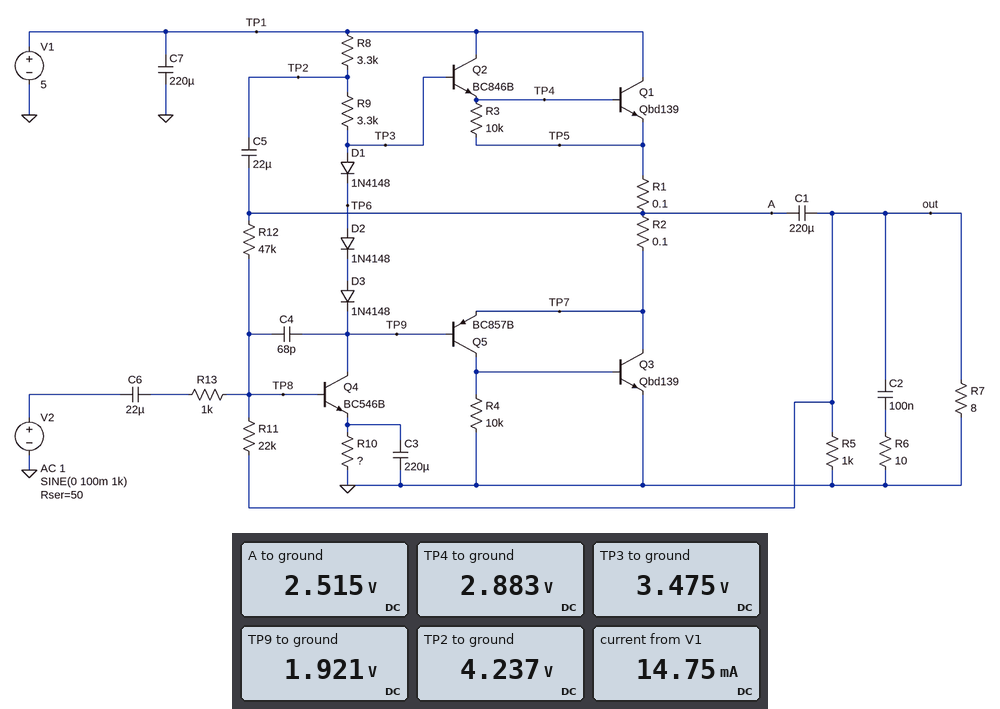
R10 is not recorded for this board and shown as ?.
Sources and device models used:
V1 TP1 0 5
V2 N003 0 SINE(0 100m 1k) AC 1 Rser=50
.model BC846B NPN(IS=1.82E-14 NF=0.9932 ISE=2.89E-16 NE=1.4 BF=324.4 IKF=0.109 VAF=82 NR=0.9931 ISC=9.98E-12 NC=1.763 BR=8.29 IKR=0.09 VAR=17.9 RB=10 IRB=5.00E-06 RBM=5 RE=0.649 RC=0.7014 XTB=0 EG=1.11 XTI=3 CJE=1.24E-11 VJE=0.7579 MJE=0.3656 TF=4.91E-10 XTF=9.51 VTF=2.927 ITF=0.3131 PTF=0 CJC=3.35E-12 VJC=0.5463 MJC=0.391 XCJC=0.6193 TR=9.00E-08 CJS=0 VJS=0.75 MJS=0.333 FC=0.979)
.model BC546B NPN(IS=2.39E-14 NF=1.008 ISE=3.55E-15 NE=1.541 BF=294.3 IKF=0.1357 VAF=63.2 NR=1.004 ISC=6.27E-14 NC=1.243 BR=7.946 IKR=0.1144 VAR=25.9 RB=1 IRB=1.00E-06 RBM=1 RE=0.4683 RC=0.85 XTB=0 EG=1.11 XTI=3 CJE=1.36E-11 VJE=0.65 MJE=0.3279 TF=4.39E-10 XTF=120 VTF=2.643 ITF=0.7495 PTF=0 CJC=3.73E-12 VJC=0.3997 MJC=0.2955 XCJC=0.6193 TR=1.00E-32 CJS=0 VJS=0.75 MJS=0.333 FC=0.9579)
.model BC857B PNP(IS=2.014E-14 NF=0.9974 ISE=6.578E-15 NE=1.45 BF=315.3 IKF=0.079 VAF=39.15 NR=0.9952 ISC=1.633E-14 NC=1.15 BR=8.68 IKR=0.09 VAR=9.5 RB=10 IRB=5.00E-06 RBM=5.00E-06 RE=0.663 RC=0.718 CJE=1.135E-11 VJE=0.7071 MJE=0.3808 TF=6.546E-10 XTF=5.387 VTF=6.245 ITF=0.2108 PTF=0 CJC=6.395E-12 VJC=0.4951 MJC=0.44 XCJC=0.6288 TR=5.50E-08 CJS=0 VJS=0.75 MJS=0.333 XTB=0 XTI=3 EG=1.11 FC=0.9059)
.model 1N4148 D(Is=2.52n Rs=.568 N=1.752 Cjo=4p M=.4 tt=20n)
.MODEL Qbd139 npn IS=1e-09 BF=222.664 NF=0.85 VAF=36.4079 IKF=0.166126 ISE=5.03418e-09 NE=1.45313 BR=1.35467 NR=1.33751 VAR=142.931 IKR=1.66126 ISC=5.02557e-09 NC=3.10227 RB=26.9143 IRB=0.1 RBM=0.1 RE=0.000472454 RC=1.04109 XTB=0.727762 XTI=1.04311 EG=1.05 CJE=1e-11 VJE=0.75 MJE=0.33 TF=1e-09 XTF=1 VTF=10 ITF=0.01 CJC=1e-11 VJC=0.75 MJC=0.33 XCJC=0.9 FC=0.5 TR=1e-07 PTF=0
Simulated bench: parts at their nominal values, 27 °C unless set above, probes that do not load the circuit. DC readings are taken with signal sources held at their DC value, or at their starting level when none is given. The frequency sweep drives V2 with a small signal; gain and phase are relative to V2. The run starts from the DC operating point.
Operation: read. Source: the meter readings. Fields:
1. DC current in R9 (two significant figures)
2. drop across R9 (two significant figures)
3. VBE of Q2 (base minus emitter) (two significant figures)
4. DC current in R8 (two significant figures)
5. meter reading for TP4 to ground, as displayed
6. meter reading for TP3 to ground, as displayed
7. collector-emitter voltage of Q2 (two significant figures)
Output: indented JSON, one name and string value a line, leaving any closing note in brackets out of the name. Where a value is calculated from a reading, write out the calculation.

{
  "DC current in R9": "(4.237 V - 3.475 V) / 3.3 kΩ = 230 µA",
  "drop across R9": "4.237 V - 3.475 V = 760 mV",
  "VBE of Q2 (base minus emitter)": "3.475 V - 2.883 V = 590 mV",
  "DC current in R8": "(5 V - 4.237 V) / 3.3 kΩ = 230 µA",
  "meter reading for TP4 to ground, as displayed": "2.883 V",
  "meter reading for TP3 to ground, as displayed": "3.475 V",
  "collector-emitter voltage of Q2": "5 V - 2.883 V = 2.1 V"
}
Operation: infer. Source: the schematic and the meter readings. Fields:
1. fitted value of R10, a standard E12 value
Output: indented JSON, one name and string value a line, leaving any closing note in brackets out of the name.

{
  "fitted value of R10, a standard E12 value": "820 Ω"
}
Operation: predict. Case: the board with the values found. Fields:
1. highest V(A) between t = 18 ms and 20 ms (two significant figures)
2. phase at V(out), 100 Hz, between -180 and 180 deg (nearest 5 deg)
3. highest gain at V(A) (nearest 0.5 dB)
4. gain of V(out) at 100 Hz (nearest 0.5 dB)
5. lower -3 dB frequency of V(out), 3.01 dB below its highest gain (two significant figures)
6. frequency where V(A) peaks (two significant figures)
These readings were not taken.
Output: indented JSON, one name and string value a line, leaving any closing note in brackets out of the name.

{
  "highest V(A) between t = 18 ms and 20 ms": "3.8 V",
  "phase at V(out), 100 Hz, between -180 and 180 deg": "-160 deg",
  "highest gain at V(A)": "31.0 dB",
  "gain of V(out) at 100 Hz": "22.0 dB",
  "lower -3 dB frequency of V(out), 3.01 dB below its highest gain": "28 Hz",
  "frequency where V(A) peaks": "17 Hz"
}
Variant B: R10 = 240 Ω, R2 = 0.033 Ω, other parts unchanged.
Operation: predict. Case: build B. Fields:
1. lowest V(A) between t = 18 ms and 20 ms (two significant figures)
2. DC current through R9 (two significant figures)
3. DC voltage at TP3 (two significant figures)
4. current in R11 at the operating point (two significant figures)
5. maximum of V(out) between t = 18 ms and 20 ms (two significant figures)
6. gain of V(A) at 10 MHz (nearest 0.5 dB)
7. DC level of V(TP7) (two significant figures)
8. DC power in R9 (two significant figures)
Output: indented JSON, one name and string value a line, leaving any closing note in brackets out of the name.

{
  "lowest V(A) between t = 18 ms and 20 ms": "820 mV",
  "DC current through R9": "280 µA",
  "DC voltage at TP3": "3.1 V",
  "current in R11 at the operating point": "31 µA",
  "maximum of V(out) between t = 18 ms and 20 ms": "1.3 V",
  "gain of V(A) at 10 MHz": "-21.0 dB",
  "DC level of V(TP7)": "2.2 V",
  "DC power in R9": "260 µW"
}
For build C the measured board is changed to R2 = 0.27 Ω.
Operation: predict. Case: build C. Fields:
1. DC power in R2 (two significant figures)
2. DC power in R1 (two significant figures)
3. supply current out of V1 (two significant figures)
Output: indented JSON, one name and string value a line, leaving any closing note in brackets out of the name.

{
  "DC power in R2": "53 µW",
  "DC power in R1": "20 µW",
  "supply current out of V1": "14 mA"
}
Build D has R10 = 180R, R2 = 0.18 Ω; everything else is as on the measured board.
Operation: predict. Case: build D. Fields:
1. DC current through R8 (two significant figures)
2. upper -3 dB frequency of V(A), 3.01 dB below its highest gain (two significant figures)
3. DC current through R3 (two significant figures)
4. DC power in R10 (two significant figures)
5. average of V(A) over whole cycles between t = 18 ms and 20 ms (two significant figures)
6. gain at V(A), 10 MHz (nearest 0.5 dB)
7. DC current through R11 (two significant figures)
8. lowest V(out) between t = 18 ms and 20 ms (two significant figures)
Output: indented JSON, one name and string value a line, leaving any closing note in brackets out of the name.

{
  "DC current through R8": "290 µA",
  "upper -3 dB frequency of V(A), 3.01 dB below its highest gain": "48 Hz",
  "DC current through R3": "38 µA",
  "DC power in R10": "15 µW",
  "average of V(A) over whole cycles between t = 18 ms and 20 ms": "2.1 V",
  "gain at V(A), 10 MHz": "-21.0 dB",
  "DC current through R11": "30 µA",
  "lowest V(out) between t = 18 ms and 20 ms": "-1.3 V"
}
